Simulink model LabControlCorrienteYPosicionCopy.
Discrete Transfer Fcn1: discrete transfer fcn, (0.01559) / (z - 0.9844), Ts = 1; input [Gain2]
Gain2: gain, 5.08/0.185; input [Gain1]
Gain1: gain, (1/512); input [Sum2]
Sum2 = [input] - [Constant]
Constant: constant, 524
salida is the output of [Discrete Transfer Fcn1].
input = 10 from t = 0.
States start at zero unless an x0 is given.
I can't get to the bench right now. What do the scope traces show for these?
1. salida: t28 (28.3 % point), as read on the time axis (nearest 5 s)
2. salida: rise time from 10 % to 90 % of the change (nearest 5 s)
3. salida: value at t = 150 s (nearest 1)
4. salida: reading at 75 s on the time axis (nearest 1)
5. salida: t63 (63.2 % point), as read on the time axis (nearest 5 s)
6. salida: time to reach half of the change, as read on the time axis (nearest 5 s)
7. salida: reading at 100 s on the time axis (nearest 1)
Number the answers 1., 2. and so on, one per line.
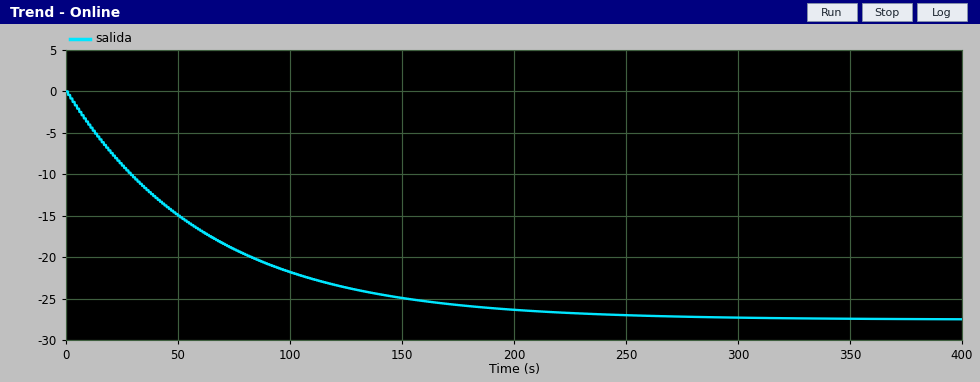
1. 20 s
2. 140 s
3. -25
4. -19
5. 65 s
6. 45 s
7. -22
